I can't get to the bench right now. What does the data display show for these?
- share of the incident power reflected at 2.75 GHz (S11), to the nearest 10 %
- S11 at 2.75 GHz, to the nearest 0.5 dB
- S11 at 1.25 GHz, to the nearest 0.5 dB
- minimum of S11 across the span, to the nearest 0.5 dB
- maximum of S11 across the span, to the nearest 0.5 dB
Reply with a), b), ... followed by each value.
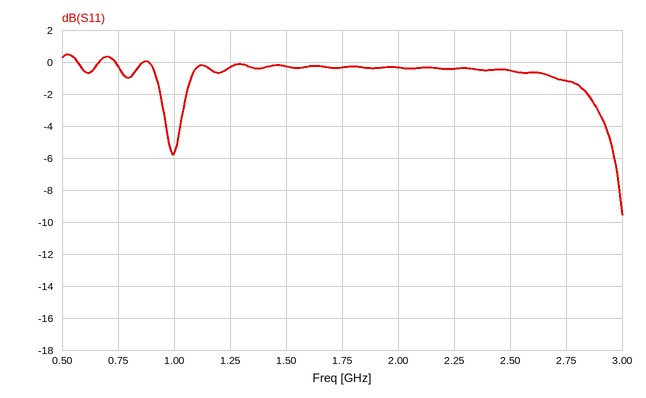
a) 80 %
b) -1.0 dB
c) -0.5 dB
d) -9.5 dB
e) 0.5 dB
